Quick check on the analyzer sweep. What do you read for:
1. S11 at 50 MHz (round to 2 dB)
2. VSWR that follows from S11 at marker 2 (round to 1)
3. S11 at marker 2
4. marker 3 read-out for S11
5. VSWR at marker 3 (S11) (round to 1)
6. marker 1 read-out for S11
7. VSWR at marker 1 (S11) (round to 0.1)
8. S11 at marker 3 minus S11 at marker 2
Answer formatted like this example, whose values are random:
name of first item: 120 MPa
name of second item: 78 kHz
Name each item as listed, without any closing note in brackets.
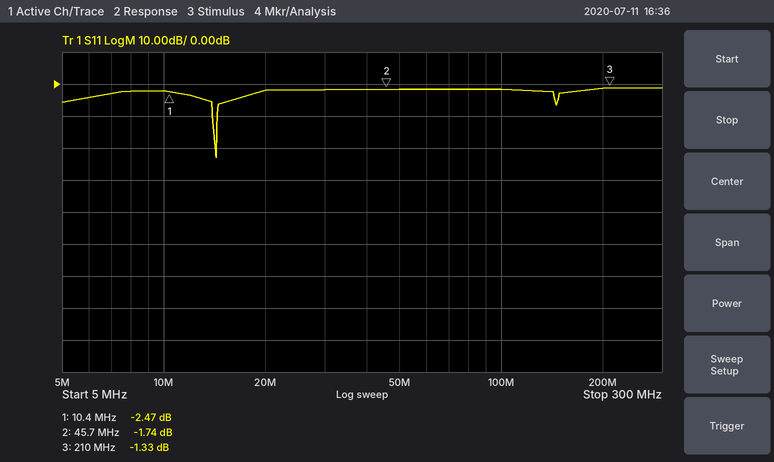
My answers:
S11 at 50 MHz: -2 dB
VSWR that follows from S11 at marker 2: 10
S11 at marker 2: -1.74 dB
marker 3 read-out for S11: -1.33 dB
VSWR at marker 3 (S11): 13
marker 1 read-out for S11: -2.47 dB
VSWR at marker 1 (S11): 7.1
S11 at marker 3 minus S11 at marker 2: 0.41 dB
